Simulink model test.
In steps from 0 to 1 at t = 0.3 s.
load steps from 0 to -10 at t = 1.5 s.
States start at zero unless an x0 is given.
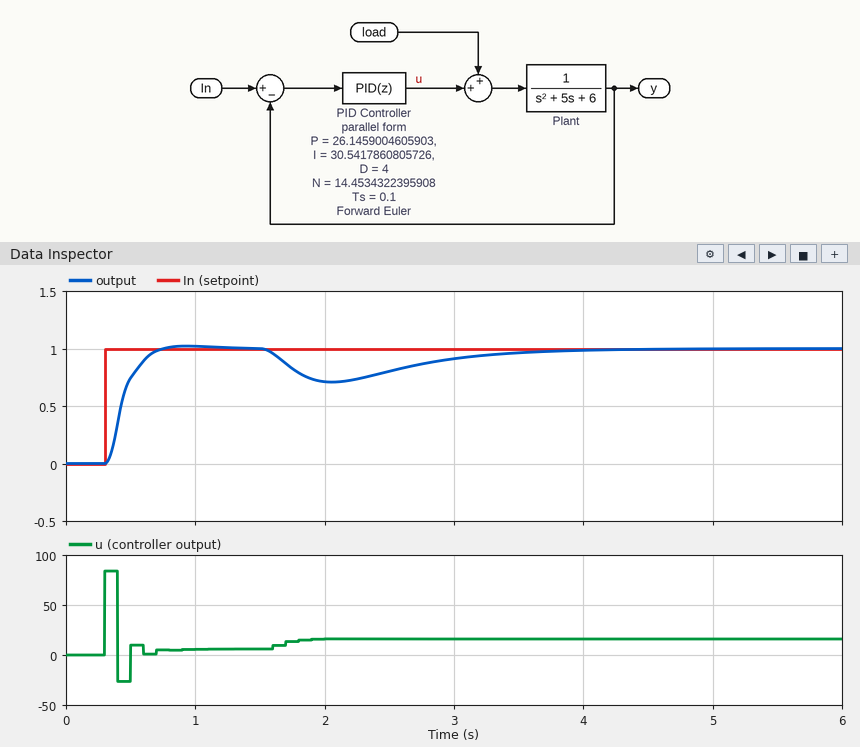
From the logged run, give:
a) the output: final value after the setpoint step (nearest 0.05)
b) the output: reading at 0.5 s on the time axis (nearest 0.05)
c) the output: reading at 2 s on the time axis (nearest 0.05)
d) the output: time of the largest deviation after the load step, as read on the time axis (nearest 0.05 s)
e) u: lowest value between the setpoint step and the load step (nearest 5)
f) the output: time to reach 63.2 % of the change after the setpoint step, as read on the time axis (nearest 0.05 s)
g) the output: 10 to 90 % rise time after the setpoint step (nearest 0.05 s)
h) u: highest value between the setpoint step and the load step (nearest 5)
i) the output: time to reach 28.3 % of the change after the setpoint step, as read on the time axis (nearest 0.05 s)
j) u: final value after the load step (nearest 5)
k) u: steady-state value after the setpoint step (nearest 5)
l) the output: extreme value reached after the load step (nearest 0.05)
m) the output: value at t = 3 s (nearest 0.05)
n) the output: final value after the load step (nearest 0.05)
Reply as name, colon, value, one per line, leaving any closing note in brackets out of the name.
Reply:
the output: final value after the setpoint step: 1.00
the output: reading at 0.5 s on the time axis: 0.75
the output: reading at 2 s on the time axis: 0.70
the output: time of the largest deviation after the load step, as read on the time axis: 2.05 s
u: lowest value between the setpoint step and the load step: -25
the output: time to reach 63.2 % of the change after the setpoint step, as read on the time axis: 0.45 s
the output: 10 to 90 % rise time after the setpoint step: 0.25 s
u: highest value between the setpoint step and the load step: 85
the output: time to reach 28.3 % of the change after the setpoint step, as read on the time axis: 0.40 s
u: final value after the load step: 15
u: steady-state value after the setpoint step: 5
the output: extreme value reached after the load step: 0.70
the output: value at t = 3 s: 0.90
the output: final value after the load step: 1.00
